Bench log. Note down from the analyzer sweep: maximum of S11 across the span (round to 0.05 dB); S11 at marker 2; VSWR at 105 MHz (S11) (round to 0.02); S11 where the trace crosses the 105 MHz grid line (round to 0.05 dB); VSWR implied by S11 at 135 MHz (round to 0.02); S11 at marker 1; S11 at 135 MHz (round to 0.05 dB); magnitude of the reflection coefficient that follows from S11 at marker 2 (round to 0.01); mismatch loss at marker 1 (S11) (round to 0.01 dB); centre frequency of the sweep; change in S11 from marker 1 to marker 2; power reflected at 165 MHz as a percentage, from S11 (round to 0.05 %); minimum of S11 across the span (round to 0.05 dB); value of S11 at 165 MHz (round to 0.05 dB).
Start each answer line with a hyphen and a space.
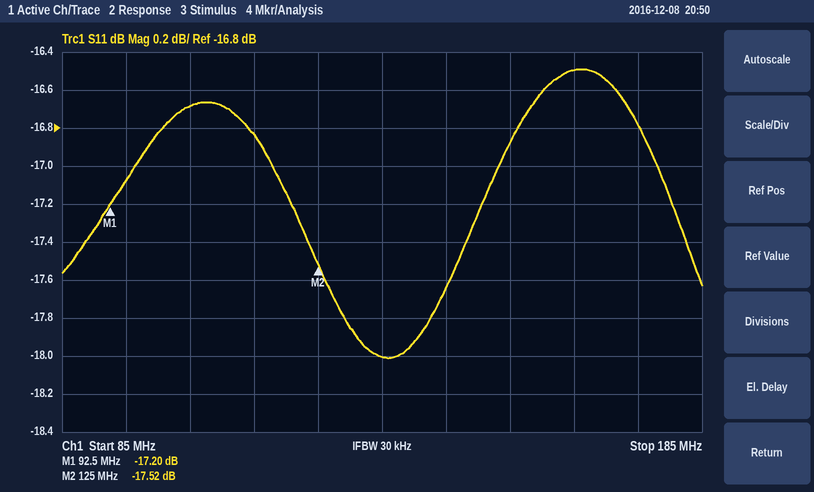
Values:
- -16.50 dB
- -17.52 dB
- 1.34
- -16.70 dB
- 1.28
- -17.20 dB
- -18.00 dB
- 0.13
- 0.08 dB
- 135 MHz
- -0.32 dB
- 2.25 %
- -18.00 dB
- -16.50 dB
